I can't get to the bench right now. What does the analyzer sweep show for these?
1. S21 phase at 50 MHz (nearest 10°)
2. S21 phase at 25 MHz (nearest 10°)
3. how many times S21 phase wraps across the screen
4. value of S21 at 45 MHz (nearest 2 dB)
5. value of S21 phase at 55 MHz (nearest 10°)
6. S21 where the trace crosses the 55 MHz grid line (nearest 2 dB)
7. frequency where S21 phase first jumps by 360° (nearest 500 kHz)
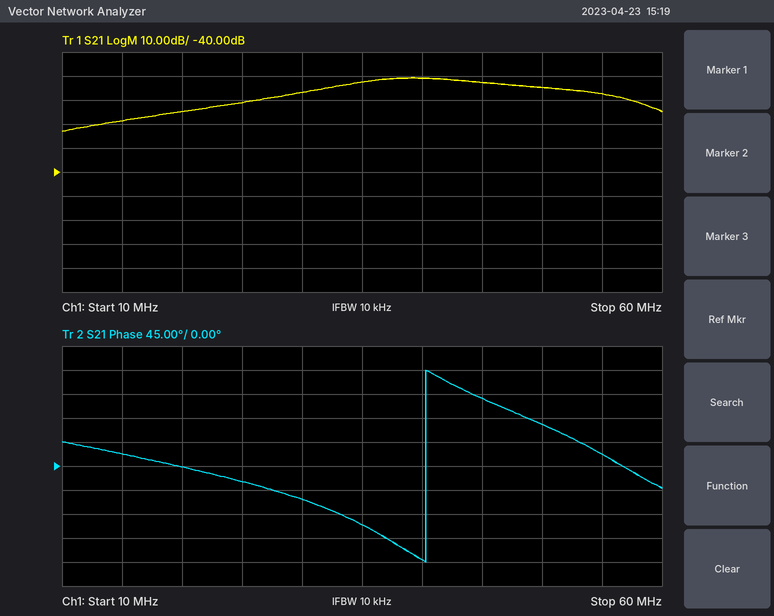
80°
-30°
1
-2 dB
20°
-8 dB
40.5 MHz
